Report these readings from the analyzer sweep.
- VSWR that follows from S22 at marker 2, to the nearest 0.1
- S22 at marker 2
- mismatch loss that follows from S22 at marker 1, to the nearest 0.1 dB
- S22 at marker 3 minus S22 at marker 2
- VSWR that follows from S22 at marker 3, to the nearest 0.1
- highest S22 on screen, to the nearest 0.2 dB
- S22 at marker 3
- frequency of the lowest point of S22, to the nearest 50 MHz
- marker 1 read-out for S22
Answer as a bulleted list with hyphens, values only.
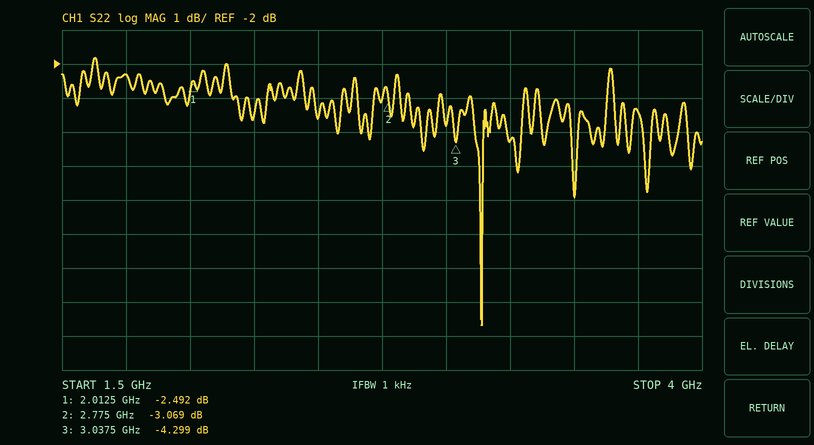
- 5.7
- -3.069 dB
- 3.6 dB
- -1.230 dB
- 4.1
- -1.8 dB
- -4.299 dB
- 3.15 GHz
- -2.492 dB
